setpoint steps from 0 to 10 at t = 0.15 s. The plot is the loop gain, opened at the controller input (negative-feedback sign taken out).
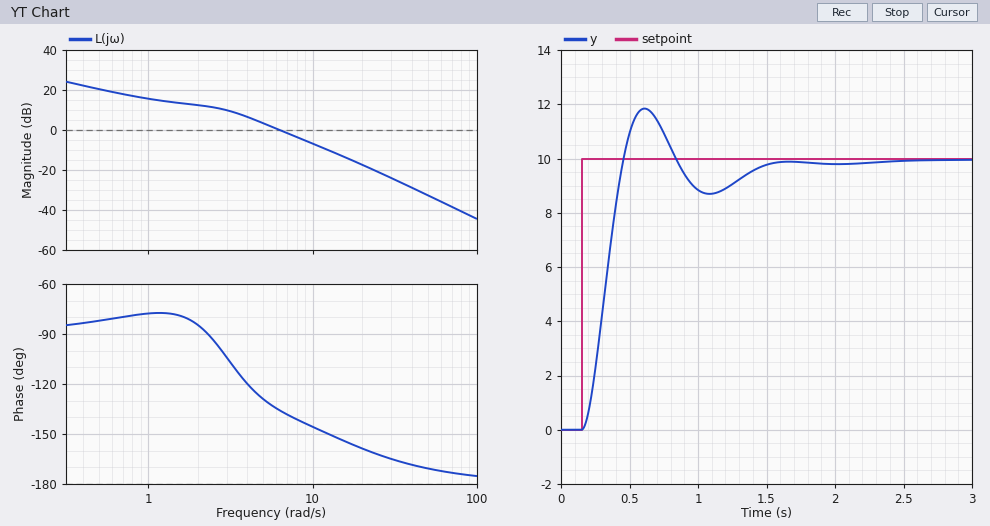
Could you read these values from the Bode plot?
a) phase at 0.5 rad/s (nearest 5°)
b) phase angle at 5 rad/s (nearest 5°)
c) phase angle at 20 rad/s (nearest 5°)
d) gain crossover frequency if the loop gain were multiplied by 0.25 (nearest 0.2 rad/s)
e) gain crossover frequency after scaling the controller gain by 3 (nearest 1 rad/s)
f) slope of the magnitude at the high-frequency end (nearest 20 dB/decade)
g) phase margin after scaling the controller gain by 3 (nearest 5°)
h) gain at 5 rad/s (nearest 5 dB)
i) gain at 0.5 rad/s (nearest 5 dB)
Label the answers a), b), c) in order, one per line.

a) -80°
b) -130°
c) -160°
d) 2.2 rad/s
e) 12 rad/s
f) -40 dB/decade
g) 30°
h) 5 dB
i) 20 dB
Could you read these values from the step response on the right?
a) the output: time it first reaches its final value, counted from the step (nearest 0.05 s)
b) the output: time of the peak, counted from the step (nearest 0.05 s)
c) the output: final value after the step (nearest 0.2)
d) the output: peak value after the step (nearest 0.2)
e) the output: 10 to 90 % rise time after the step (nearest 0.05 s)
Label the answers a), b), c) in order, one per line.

a) 0.30 s
b) 0.45 s
c) 10.0
d) 11.8
e) 0.20 s
